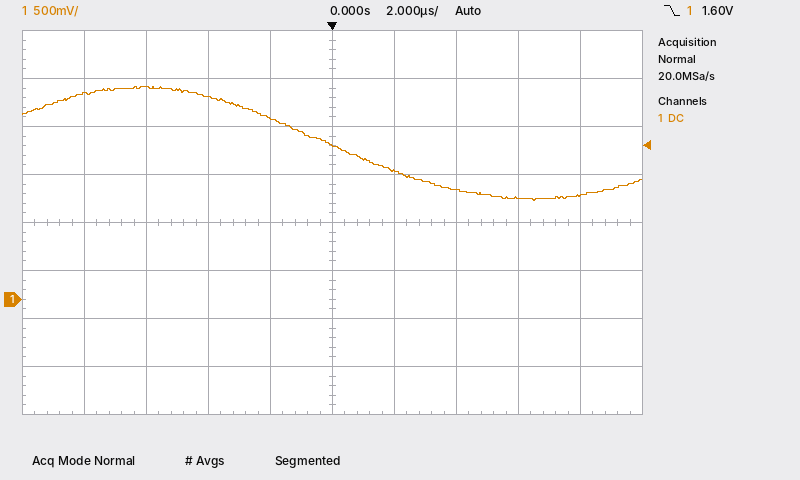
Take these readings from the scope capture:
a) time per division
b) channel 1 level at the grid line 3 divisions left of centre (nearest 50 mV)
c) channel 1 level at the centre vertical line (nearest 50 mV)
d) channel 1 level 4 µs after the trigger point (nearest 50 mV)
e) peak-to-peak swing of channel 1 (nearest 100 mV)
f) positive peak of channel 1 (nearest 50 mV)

2 µs
2.20 V
1.60 V
1.15 V
1.20 V
2.20 V
